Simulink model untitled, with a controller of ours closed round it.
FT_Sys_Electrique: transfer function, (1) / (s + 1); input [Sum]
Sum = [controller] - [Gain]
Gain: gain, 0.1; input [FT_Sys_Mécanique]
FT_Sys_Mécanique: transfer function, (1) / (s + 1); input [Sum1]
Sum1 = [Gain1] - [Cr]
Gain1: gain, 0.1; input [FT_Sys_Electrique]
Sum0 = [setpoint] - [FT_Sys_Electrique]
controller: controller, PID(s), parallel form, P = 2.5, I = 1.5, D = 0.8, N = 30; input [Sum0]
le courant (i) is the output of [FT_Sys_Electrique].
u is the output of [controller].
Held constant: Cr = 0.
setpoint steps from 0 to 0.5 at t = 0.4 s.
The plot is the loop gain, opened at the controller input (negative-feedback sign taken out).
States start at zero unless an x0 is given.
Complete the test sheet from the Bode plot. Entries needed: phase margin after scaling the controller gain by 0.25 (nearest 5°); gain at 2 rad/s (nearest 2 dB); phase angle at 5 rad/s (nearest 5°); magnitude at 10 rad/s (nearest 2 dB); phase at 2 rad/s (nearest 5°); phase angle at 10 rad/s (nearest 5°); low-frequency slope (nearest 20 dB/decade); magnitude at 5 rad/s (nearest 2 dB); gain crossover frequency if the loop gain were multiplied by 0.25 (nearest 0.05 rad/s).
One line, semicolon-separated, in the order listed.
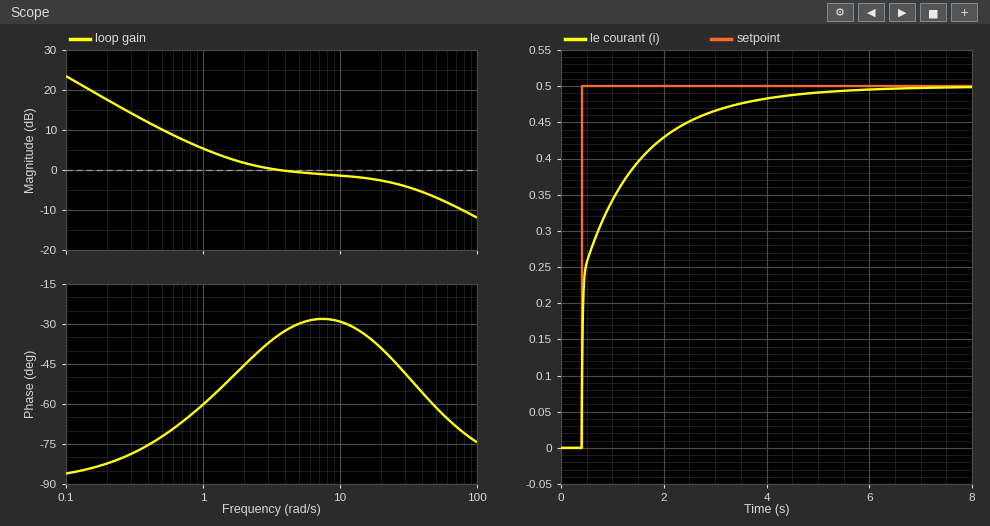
105°; 2 dB; -30°; -2 dB; -45°; -30°; -20 dB/decade; 0 dB; 0.40 rad/s
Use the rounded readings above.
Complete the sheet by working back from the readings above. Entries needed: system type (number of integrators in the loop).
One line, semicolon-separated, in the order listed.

1
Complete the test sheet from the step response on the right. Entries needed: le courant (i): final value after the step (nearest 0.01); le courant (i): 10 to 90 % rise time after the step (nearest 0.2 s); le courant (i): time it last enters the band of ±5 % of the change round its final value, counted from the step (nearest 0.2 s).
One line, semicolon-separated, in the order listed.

0.50; 2.0 s; 3.0 s
